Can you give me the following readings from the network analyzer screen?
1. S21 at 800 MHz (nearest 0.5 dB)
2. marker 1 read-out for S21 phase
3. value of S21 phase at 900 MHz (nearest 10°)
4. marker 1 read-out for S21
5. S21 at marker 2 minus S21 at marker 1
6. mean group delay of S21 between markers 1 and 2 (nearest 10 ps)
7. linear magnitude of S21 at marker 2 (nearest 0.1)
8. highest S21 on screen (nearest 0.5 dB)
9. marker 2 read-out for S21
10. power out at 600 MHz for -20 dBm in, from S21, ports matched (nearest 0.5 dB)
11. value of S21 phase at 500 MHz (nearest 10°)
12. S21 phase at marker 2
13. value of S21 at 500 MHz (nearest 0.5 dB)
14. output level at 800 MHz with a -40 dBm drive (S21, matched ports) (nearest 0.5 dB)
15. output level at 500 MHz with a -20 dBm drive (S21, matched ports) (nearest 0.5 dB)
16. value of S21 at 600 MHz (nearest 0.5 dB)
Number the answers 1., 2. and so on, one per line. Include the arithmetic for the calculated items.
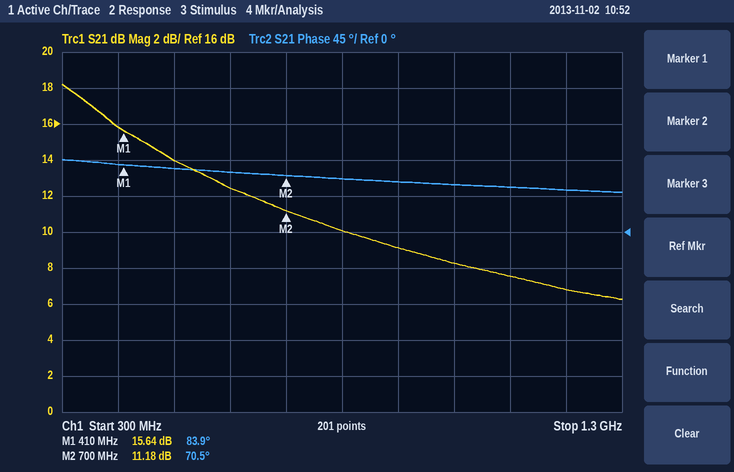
1. 10.0 dB
2. 83.9°
3. 60°
4. 15.64 dB
5. 11.18 − (15.64) = -4.46 dB
6. −(70.5° − (83.9°))/(360° × 290 MHz) ≈ 128 ps, so 130 ps to the nearest 10 ps
7. 10^(11.18/20) ≈ 3.6
8. 18.0 dB
9. 11.18 dB
10. -20 dBm + (12.5 dB) = -7.5 dBm
11. 80°
12. 70.5°
13. 14.0 dB
14. -40 dBm + (10.0 dB) = -30.0 dBm
15. -20 dBm + (14.0 dB) = -6.0 dBm
16. 12.5 dB
